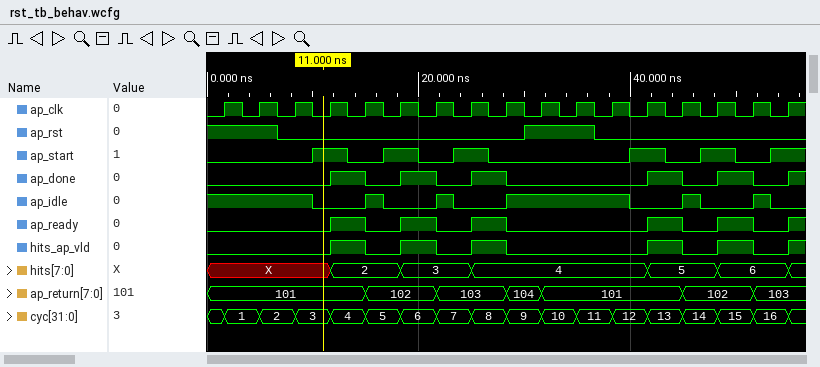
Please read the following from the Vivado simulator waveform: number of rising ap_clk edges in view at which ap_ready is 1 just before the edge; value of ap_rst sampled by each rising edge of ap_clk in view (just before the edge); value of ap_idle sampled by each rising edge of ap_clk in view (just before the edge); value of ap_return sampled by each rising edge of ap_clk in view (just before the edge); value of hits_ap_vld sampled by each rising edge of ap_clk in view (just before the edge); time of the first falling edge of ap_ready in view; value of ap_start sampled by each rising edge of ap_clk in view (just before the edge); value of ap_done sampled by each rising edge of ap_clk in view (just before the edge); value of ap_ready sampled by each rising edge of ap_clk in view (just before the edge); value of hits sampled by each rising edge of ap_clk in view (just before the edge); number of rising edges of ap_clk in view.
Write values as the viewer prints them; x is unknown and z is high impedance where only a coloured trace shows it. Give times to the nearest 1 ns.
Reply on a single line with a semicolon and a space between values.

5; 1 1 0 0 0 0 0 0 0 1 1 0 0 0 0 0 0; 1 1 1 0 0 0 0 0 0 1 1 1 0 0 0 0 0; 101, 101, 101, 101, 101, 102, 102, 103, 103, 104, 101, 101, 101, 101, 102, 102, 103; 0 0 0 0 1 0 1 0 1 0 0 0 0 1 0 1 0; 15 ns; 0 0 0 1 0 1 0 1 0 0 0 0 1 0 1 0 1; 0 0 0 0 1 0 1 0 1 0 0 0 0 1 0 1 0; 0 0 0 0 1 0 1 0 1 0 0 0 0 1 0 1 0; X, X, X, X, 2, 2, 3, 3, 4, 4, 4, 4, 4, 5, 5, 6, 6; 17
